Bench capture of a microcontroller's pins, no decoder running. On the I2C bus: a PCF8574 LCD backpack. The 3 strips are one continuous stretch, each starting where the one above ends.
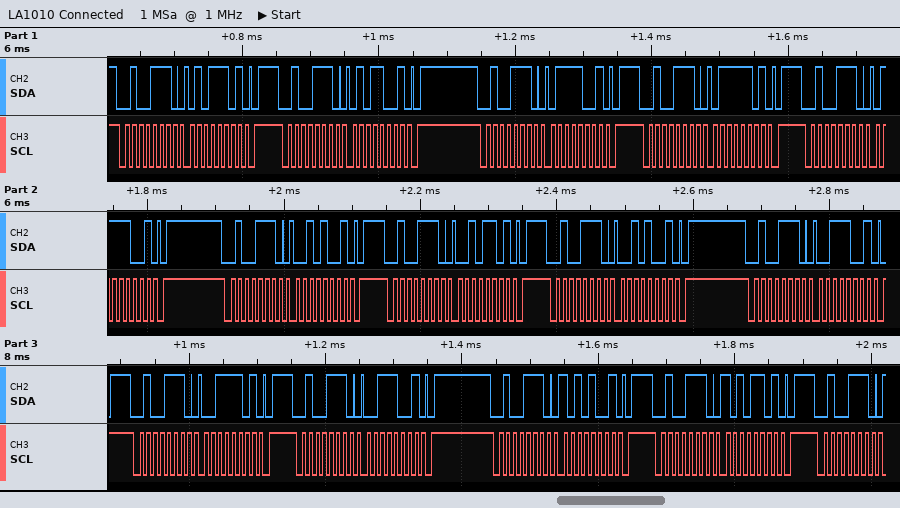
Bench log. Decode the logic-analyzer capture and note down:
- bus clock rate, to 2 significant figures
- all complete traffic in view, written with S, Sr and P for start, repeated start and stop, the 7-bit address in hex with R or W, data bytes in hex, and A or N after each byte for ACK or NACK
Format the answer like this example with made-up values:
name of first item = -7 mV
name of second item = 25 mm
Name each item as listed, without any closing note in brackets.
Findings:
bus clock rate, to 2 significant figures = 100 kHz
all complete traffic in view, written with S, Sr and P for start, repeated start and stop, the 7-bit address in hex with R or W, data bytes in hex, and A or N after each byte for ACK or NACK = S 27W A 5D A P S 27W A 59 A P S 27W A 79 A P S 27W A 7D A P S 27W A 79 A P S 27W A 29 A P S 27W A 2D A P S 27W A 29 A P S 27W A 39 A P S 27W A 3D A P S 27W A 39 A P S 27W A A9 A P S 27W A AD A P S 27W A
